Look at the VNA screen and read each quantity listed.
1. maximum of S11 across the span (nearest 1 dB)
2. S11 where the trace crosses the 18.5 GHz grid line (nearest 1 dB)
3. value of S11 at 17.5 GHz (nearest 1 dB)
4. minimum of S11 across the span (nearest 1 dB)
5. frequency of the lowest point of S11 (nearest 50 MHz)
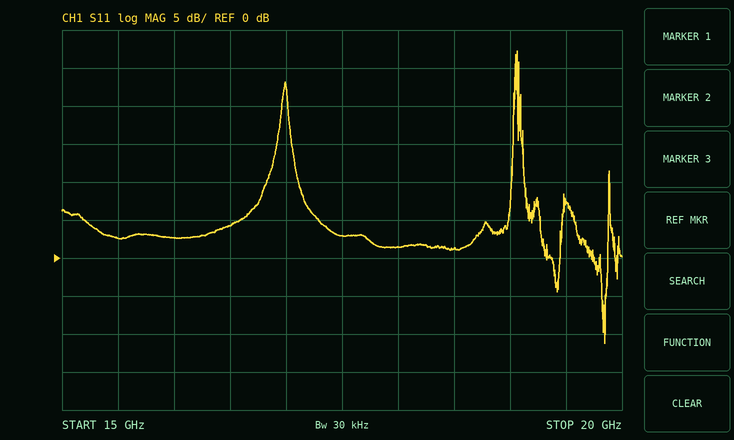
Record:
27 dB
1 dB
3 dB
-11 dB
19.85 GHz
